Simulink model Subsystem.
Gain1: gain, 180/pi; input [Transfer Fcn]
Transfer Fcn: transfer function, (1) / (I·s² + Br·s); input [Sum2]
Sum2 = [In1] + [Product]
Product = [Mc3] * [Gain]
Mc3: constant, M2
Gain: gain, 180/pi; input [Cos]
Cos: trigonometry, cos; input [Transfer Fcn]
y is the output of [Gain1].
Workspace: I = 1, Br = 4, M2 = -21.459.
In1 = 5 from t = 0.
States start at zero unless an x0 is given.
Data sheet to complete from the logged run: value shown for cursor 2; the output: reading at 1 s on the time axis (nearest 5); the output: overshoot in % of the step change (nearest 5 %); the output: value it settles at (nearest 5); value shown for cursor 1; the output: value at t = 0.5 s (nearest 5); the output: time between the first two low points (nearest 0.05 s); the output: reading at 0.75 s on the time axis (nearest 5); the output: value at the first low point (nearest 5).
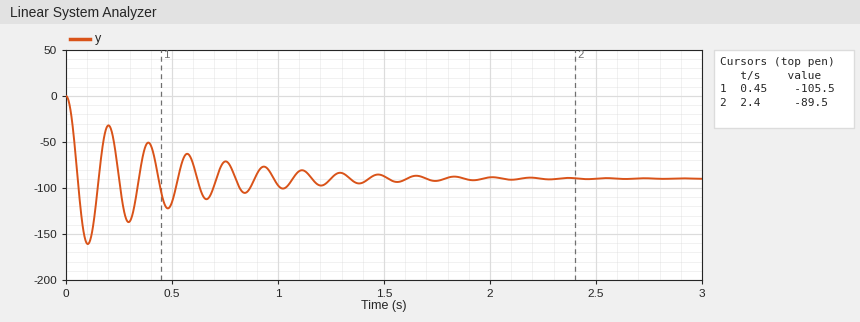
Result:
-89.5
-95
80 %
-90
-105.5
-115
0.20 s
-70
-160
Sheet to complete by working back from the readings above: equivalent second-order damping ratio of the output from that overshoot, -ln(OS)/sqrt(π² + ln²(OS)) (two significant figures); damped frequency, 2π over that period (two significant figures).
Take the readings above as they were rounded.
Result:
0.071
31 rad/s
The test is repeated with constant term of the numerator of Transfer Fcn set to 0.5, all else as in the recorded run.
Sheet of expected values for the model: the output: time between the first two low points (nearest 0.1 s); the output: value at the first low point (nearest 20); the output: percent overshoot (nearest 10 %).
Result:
0.3 s
-160
70 %
